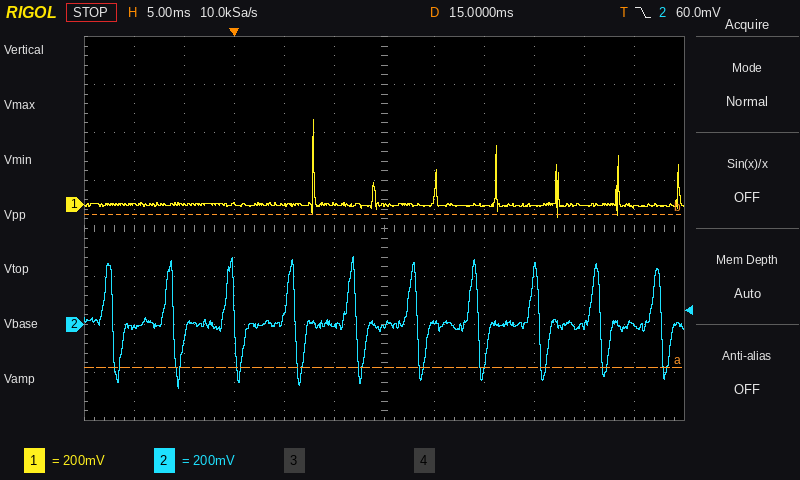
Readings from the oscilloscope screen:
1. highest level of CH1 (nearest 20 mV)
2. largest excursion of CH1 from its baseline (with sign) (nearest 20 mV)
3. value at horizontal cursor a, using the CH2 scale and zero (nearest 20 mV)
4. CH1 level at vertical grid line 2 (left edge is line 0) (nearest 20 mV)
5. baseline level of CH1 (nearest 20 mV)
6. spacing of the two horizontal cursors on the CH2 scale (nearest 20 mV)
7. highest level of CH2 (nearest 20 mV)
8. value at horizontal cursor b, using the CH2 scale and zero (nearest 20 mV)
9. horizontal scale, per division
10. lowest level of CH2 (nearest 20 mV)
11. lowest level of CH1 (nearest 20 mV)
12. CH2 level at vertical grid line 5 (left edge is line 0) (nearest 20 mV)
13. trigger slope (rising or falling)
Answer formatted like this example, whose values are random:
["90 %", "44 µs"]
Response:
["360 mV", "+360 mV", "-180 mV", "0 mV", "0 mV", "640 mV", "280 mV", "460 mV", "5 ms", "-260 mV", "-60 mV", "0 mV", "falling"]
